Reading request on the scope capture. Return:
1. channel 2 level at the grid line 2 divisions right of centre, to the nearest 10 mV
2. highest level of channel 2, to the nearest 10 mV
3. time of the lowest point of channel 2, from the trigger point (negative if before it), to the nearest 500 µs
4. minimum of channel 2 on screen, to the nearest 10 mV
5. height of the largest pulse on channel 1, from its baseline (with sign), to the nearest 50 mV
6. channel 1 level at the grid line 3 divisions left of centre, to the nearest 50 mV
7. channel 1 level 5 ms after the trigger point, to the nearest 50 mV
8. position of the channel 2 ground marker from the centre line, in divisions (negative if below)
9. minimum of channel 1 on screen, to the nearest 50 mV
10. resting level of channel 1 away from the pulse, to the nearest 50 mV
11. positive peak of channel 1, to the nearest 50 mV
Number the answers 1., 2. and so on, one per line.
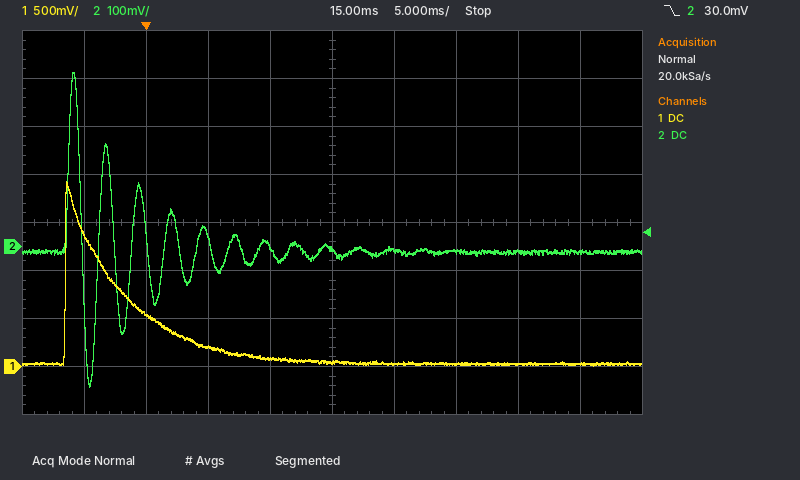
1. -10 mV
2. 360 mV
3. -4.5 ms
4. -290 mV
5. +1.90 V
6. 550 mV
7. 200 mV
8. -0.5 div
9. 0 mV
10. 50 mV
11. 1.95 V
